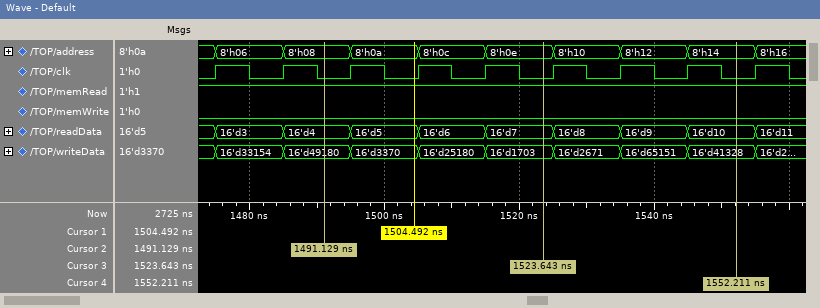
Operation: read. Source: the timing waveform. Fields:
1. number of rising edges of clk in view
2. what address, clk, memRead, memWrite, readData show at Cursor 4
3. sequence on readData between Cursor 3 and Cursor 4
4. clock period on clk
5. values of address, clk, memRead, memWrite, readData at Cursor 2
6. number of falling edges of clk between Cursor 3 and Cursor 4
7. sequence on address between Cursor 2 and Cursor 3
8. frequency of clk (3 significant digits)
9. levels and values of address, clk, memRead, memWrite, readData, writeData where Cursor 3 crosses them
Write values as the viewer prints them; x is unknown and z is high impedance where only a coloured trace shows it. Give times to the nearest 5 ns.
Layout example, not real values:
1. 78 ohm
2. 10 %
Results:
1. 9
2. address=8'h14, clk=0, memRead=1, memWrite=0, readData=16'd10
3. 16'd7, 16'd8, 16'd9, 16'd10
4. 10 ns
5. address=8'h08, clk=0, memRead=1, memWrite=0, readData=16'd4
6. 3
7. 8'h08, 8'h0a, 8'h0c, 8'h0e
8. 100 MHz
9. address=8'h0e, clk=0, memRead=1, memWrite=0, readData=16'd7, writeData=16'd1703
